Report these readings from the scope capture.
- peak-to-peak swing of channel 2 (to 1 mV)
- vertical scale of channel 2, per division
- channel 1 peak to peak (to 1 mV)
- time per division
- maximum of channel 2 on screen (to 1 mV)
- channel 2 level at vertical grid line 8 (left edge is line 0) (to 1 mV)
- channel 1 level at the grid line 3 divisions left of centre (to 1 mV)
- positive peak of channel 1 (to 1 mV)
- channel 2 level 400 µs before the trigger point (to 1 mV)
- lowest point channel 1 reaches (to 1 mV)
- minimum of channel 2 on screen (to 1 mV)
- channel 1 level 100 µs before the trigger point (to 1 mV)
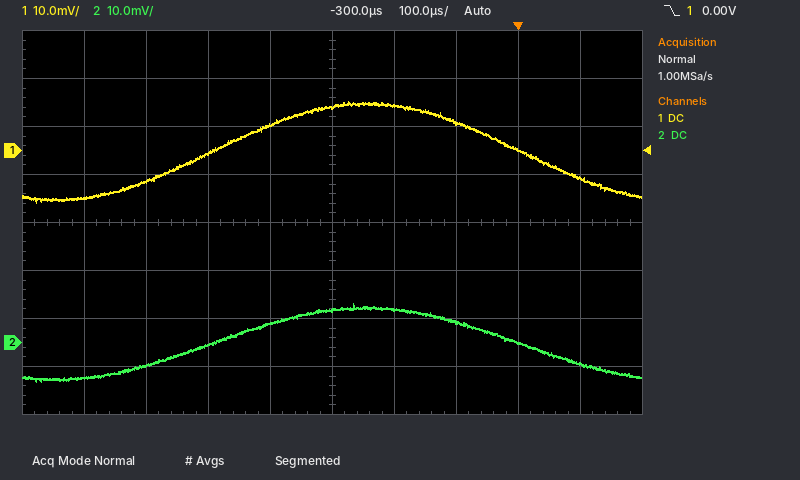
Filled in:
16 mV
10 mV
21 mV
100 µs
8 mV
0 mV
-6 mV
10 mV
4 mV
-11 mV
-8 mV
6 mV
